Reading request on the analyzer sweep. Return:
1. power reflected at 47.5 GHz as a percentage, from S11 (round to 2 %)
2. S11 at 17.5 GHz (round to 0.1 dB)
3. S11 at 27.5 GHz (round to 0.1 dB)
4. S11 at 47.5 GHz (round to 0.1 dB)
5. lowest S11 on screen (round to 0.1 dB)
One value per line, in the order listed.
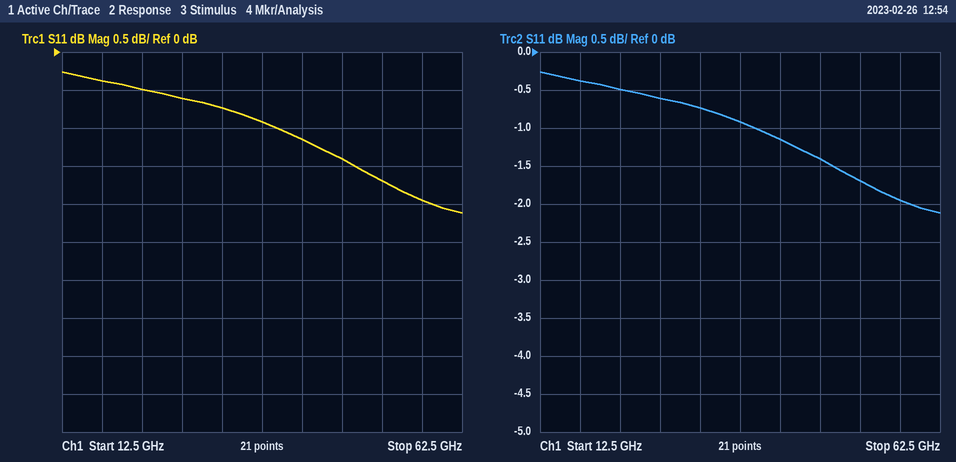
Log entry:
72 %
-0.4 dB
-0.6 dB
-1.4 dB
-2.1 dB
